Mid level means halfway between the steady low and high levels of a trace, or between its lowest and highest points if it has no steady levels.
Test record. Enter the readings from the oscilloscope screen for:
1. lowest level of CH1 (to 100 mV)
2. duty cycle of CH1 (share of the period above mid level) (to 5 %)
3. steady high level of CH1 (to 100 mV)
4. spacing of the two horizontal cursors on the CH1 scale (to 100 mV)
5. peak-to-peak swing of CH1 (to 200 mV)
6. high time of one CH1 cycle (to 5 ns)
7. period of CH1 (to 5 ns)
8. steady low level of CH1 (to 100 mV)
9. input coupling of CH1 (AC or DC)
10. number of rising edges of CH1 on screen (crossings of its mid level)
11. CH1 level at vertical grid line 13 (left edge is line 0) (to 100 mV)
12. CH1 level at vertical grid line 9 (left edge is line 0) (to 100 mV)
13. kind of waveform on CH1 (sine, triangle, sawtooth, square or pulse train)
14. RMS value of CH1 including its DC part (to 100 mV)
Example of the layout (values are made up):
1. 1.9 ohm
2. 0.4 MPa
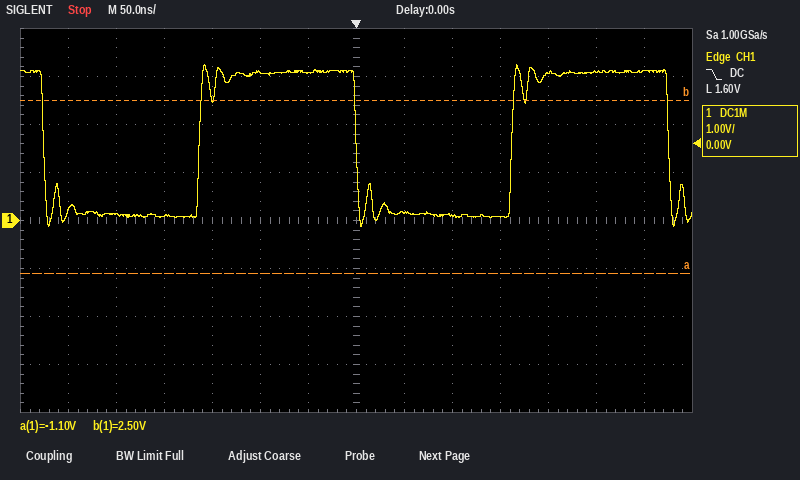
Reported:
1. -100 mV
2. 50 %
3. 3.1 V
4. 3.6 V
5. 3.4 V
6. 165 ns
7. 325 ns
8. 100 mV
9. DC
10. 2
11. 3.1 V
12. 100 mV
13. square
14. 2.2 V
